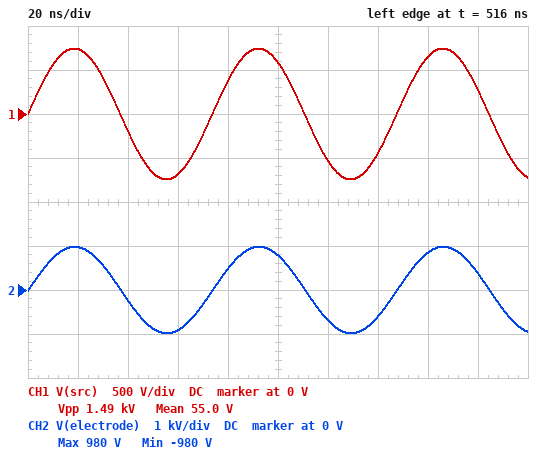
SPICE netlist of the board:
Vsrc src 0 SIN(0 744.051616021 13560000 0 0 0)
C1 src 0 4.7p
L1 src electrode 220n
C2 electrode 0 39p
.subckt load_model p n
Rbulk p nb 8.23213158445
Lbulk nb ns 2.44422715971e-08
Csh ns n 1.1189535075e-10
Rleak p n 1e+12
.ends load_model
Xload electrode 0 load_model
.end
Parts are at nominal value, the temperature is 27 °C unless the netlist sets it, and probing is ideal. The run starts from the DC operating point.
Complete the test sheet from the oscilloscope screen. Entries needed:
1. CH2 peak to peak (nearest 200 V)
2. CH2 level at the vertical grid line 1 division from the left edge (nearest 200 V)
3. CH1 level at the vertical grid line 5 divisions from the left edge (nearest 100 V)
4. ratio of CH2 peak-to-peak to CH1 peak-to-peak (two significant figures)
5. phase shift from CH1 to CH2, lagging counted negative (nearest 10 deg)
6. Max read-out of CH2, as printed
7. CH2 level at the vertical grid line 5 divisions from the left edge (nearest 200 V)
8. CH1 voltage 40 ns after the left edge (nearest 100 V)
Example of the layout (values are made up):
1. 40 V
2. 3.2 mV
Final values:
1. 2.0 kV
2. 1.0 kV
3. 600 V
4. 1.3
5. 0 deg
6. 980 V
7. 800 V
8. -200 V
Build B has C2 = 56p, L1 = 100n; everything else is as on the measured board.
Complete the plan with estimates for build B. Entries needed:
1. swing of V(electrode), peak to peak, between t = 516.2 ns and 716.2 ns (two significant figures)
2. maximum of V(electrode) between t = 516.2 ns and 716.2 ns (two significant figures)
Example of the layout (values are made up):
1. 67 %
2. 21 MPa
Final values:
1. 1.7 kV
2. 850 V
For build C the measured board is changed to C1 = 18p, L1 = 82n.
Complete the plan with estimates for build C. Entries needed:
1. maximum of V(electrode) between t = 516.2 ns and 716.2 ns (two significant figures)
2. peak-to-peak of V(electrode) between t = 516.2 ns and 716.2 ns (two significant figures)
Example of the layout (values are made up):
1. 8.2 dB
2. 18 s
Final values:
1. 820 V
2. 1.6 kV
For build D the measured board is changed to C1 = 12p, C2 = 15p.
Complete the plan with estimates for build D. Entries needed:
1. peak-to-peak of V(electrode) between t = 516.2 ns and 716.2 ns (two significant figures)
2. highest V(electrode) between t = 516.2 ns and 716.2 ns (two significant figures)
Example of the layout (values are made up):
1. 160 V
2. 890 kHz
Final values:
1. 1.9 kV
2. 940 V
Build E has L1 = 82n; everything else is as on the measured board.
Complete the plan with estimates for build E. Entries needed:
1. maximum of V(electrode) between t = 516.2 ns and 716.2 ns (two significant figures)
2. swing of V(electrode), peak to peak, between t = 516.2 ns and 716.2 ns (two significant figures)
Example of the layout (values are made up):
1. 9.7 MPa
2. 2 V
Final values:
1. 820 V
2. 1.6 kV
